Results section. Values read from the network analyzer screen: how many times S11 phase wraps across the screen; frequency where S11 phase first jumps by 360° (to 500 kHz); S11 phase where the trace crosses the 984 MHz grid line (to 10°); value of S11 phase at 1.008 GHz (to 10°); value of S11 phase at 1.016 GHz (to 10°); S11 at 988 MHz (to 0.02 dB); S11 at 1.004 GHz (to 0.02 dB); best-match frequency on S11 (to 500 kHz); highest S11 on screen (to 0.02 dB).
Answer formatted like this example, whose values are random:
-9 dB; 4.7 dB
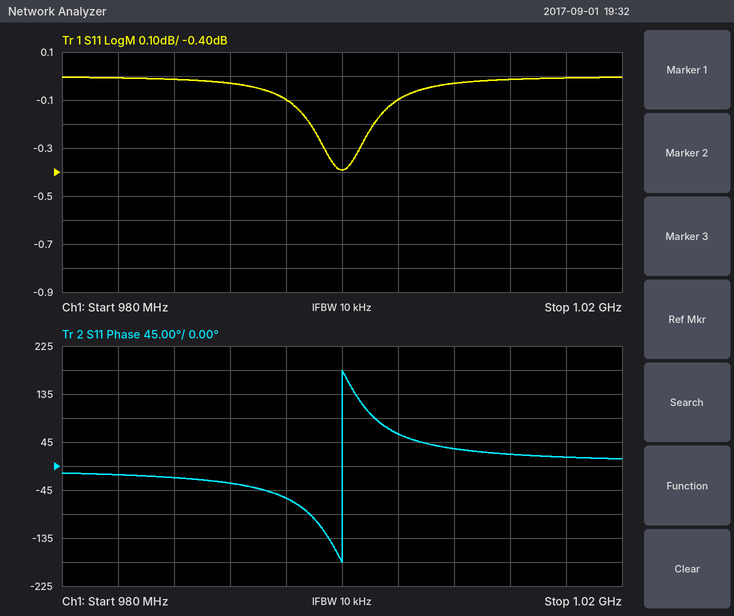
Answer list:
1; 1.0000 GHz; -20°; 30°; 20°; -0.02 dB; -0.10 dB; 1.0000 GHz; 0.00 dB
